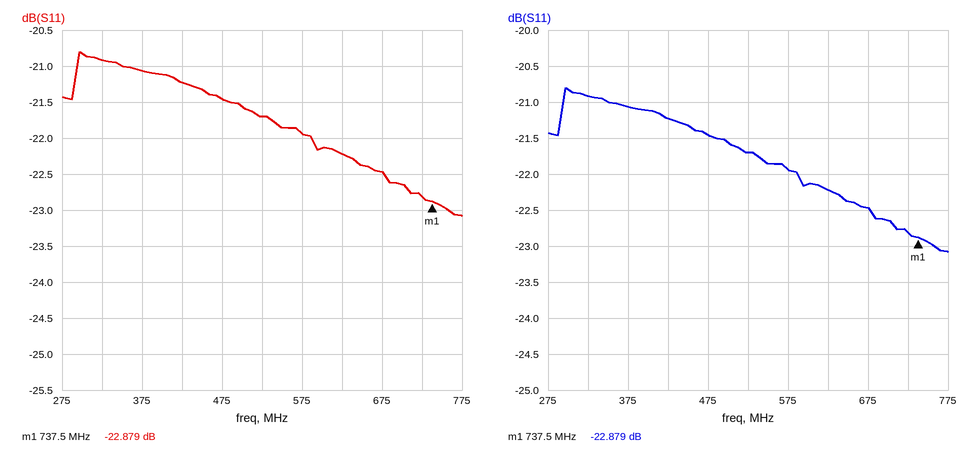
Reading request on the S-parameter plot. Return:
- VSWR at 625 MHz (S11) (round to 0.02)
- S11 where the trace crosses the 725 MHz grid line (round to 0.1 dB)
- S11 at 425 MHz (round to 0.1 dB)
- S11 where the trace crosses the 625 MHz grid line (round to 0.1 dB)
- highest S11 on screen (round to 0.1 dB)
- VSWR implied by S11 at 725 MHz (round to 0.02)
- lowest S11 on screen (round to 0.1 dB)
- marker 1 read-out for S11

1.16
-22.8 dB
-21.2 dB
-22.2 dB
-20.8 dB
1.16
-23.1 dB
-22.879 dB
